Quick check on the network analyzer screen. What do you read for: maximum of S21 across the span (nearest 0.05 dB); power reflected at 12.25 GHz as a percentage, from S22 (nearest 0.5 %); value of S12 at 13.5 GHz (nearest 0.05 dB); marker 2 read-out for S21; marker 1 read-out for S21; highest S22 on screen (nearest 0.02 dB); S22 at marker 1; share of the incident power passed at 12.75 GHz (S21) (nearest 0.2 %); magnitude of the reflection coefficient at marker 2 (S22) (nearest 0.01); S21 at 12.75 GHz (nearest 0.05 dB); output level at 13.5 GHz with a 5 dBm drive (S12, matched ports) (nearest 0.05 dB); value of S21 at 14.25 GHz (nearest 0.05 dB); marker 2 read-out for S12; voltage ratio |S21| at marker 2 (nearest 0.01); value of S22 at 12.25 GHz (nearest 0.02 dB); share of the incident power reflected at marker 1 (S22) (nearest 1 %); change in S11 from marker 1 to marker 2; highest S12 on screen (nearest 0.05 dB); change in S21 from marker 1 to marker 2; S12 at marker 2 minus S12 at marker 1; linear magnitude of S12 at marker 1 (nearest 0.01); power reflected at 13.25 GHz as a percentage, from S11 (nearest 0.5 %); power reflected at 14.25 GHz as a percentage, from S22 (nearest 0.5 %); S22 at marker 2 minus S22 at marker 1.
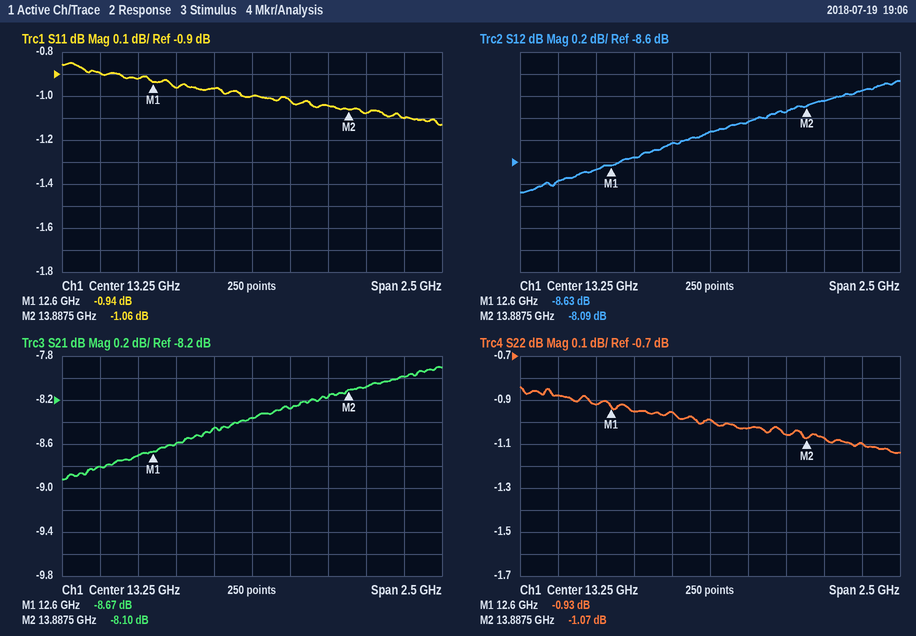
-7.90 dB
81.5 %
-8.25 dB
-8.10 dB
-8.67 dB
-0.84 dB
-0.93 dB
13.8 %
0.88
-8.60 dB
-3.25 dBm
-8.00 dB
-8.09 dB
0.39
-0.88 dB
81 %
-0.12 dB
-7.85 dB
0.57 dB
0.54 dB
0.37
79.5 %
77.5 %
-0.14 dB
